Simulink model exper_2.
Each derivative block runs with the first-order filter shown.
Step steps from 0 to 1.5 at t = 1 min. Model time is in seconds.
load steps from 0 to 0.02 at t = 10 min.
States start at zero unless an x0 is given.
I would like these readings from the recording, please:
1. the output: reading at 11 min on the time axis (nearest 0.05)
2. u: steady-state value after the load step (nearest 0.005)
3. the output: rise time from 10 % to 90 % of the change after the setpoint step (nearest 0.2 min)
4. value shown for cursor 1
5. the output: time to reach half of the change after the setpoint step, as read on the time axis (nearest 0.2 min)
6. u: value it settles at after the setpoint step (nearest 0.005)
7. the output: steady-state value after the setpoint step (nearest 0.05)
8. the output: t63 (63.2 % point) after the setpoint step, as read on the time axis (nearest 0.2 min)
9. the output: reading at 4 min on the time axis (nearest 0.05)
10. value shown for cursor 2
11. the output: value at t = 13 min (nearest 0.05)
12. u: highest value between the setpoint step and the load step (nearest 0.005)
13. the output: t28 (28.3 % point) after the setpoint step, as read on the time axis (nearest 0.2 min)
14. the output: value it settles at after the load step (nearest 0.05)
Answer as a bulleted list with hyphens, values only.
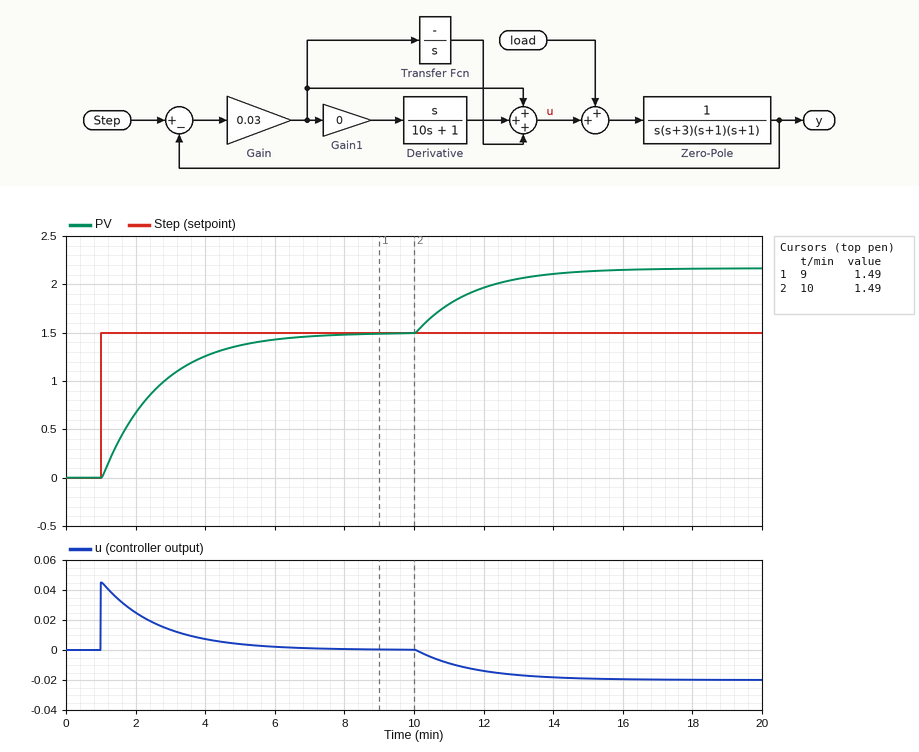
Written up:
- 1.80
- -0.020
- 3.6 min
- 1.49
- 2.2 min
- 0.000
- 1.50
- 2.6 min
- 1.25
- 1.49
- 2.05
- 0.045
- 1.6 min
- 2.15
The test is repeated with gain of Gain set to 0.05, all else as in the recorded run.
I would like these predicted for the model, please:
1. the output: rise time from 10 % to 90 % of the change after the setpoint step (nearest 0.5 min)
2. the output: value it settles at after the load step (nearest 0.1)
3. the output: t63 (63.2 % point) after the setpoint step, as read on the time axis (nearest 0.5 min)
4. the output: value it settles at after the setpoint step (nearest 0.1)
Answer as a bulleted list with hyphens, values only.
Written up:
- 2.0 min
- 1.9
- 2.0 min
- 1.5
